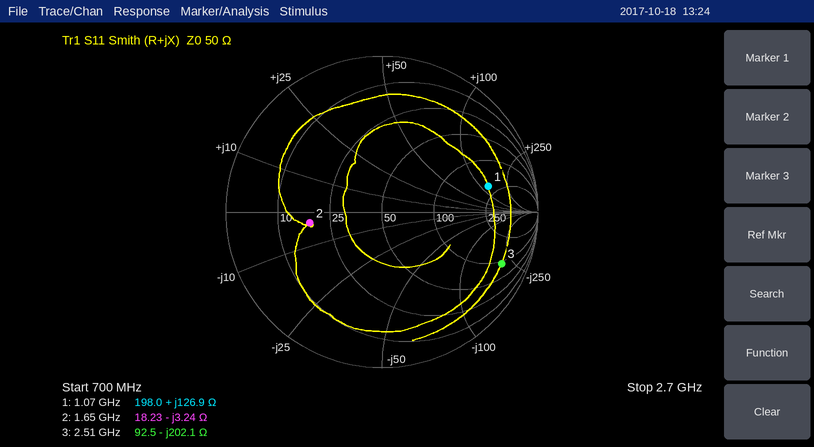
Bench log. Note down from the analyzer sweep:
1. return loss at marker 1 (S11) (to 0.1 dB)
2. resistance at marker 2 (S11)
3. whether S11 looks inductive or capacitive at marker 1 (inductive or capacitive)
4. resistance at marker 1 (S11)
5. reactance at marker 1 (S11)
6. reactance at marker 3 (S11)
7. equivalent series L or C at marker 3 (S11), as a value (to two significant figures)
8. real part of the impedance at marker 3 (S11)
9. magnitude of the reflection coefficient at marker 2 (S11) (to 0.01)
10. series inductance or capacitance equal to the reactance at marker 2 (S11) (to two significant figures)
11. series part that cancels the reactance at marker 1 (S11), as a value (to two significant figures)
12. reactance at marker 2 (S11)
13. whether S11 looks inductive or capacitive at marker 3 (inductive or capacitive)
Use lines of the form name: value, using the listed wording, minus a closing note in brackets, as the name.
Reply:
return loss at marker 1 (S11): 3.1 dB
resistance at marker 2: 18.23 Ω
whether S11 looks inductive or capacitive at marker 1: inductive
resistance at marker 1: 198.0 Ω
reactance at marker 1: +126.9 Ω
reactance at marker 3: -202.1 Ω
equivalent series L or C at marker 3 (S11), as a value: 310 fF
real part of the impedance at marker 3: 92.5 Ω
magnitude of the reflection coefficient at marker 2 (S11): 0.47
series inductance or capacitance equal to the reactance at marker 2 (S11): 30 pF
series part that cancels the reactance at marker 1 (S11), as a value: 1.2 pF
reactance at marker 2: -3.24 Ω
whether S11 looks inductive or capacitive at marker 3: capacitive
